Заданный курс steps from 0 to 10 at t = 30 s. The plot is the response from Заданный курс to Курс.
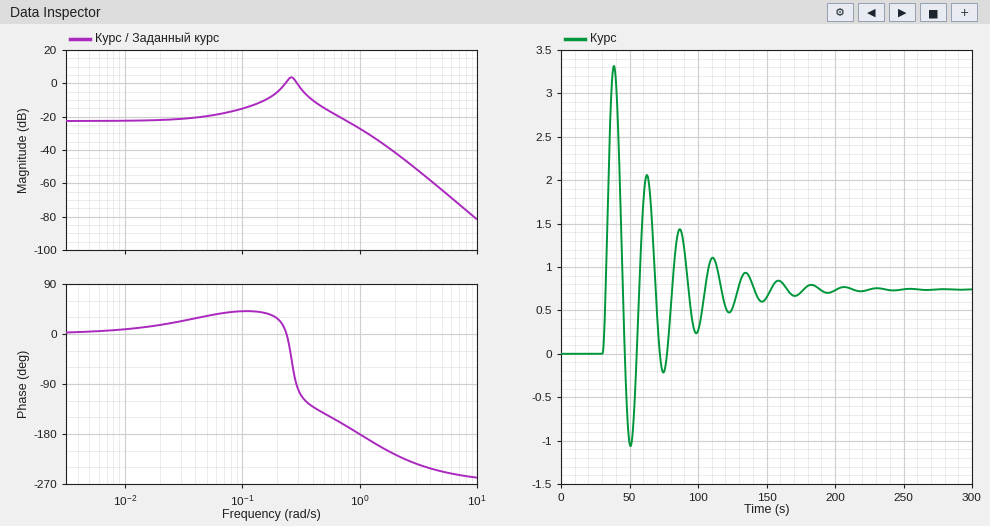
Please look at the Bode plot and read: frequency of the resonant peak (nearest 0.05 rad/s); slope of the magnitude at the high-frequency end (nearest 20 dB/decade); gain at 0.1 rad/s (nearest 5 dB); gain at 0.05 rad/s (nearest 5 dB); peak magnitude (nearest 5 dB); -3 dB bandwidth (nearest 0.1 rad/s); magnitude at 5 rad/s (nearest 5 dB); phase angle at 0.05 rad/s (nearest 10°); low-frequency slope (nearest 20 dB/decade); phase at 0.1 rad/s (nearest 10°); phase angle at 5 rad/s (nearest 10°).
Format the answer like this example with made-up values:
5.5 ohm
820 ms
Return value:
0.25 rad/s
-60 dB/decade
-15 dB
-20 dB
5 dB
0.9 rad/s
-65 dB
30°
0 dB/decade
40°
-250°
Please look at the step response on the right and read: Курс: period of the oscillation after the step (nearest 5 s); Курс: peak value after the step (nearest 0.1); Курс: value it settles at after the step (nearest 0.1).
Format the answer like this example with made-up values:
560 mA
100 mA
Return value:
25 s
3.3
0.7
